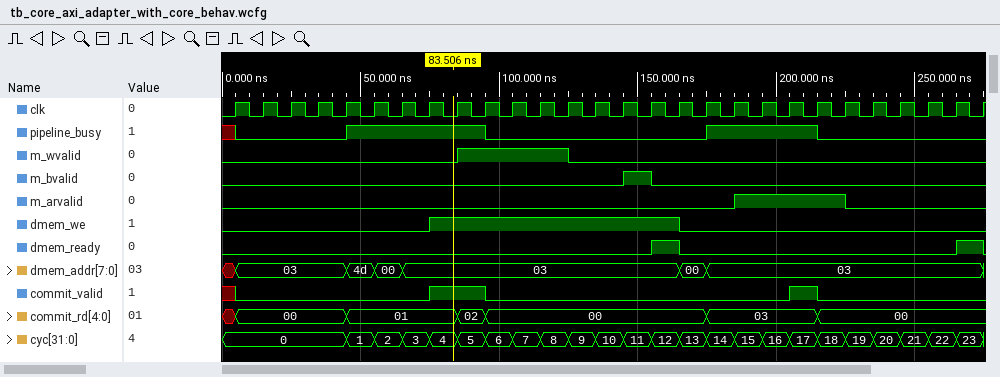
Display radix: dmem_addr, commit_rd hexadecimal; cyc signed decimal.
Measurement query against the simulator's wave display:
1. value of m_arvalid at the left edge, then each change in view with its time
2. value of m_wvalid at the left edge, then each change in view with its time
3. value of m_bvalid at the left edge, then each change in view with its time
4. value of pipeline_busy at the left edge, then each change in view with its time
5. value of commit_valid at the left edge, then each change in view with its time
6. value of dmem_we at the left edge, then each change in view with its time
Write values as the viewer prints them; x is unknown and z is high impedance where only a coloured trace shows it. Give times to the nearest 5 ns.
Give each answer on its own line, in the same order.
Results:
0, 1 at 185 ns, 0 at 225 ns
0, 1 at 85 ns, 0 at 125 ns
0, 1 at 145 ns, 0 at 155 ns
x, 0 at 5 ns, 1 at 45 ns, 0 at 95 ns, 1 at 175 ns, 0 at 215 ns
x, 0 at 5 ns, 1 at 75 ns, 0 at 95 ns, 1 at 205 ns, 0 at 215 ns
0, 1 at 75 ns, 0 at 165 ns
